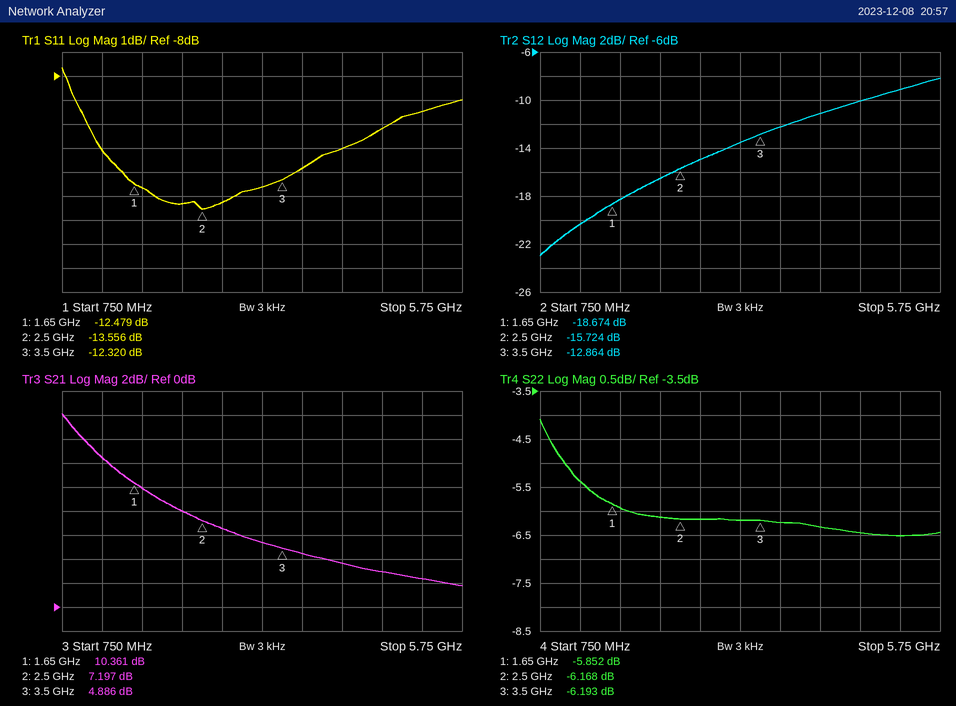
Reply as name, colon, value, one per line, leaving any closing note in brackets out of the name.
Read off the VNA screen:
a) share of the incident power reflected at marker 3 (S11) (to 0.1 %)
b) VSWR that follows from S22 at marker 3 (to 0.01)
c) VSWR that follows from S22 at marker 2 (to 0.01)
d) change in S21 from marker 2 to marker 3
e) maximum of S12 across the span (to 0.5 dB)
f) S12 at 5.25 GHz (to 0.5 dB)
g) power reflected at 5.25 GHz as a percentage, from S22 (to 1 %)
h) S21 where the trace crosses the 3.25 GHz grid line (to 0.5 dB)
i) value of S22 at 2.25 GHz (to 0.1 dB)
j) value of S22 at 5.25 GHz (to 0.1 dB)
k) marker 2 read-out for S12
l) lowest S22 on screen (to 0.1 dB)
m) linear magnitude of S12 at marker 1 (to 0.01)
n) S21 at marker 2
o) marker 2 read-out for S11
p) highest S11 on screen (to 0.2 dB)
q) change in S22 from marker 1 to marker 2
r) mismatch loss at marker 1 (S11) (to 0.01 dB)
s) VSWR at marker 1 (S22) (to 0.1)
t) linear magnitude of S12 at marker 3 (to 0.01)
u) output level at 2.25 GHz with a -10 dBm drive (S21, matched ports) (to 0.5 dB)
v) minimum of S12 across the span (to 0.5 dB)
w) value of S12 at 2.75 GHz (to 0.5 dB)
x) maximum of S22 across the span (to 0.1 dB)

share of the incident power reflected at marker 3 (S11): 5.9 %
VSWR that follows from S22 at marker 3: 2.92
VSWR that follows from S22 at marker 2: 2.93
change in S21 from marker 2 to marker 3: -2.311 dB
maximum of S12 across the span: -8.0 dB
S12 at 5.25 GHz: -9.0 dB
power reflected at 5.25 GHz as a percentage, from S22: 22 %
S21 where the trace crosses the 3.25 GHz grid line: 5.5 dB
value of S22 at 2.25 GHz: -6.1 dB
value of S22 at 5.25 GHz: -6.5 dB
marker 2 read-out for S12: -15.724 dB
lowest S22 on screen: -6.5 dB
linear magnitude of S12 at marker 1: 0.12
S21 at marker 2: 7.197 dB
marker 2 read-out for S11: -13.556 dB
highest S11 on screen: -7.6 dB
change in S22 from marker 1 to marker 2: -0.316 dB
mismatch loss at marker 1 (S11): 0.25 dB
VSWR at marker 1 (S22): 3.1
linear magnitude of S12 at marker 3: 0.23
output level at 2.25 GHz with a -10 dBm drive (S21, matched ports): -2.0 dBm
minimum of S12 across the span: -23.0 dB
value of S12 at 2.75 GHz: -15.0 dB
maximum of S22 across the span: -4.1 dB
